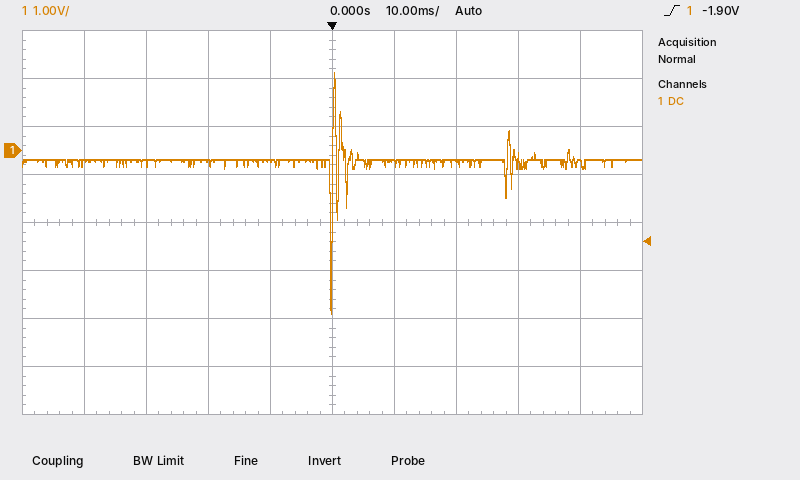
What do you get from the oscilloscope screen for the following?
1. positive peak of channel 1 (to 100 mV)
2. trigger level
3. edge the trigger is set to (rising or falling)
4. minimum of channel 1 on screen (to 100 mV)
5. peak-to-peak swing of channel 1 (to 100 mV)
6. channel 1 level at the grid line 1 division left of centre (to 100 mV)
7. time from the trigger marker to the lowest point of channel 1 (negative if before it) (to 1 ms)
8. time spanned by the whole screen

1.6 V
-1.90 V
rising
-3.4 V
5.0 V
-200 mV
0 ms
100 ms
